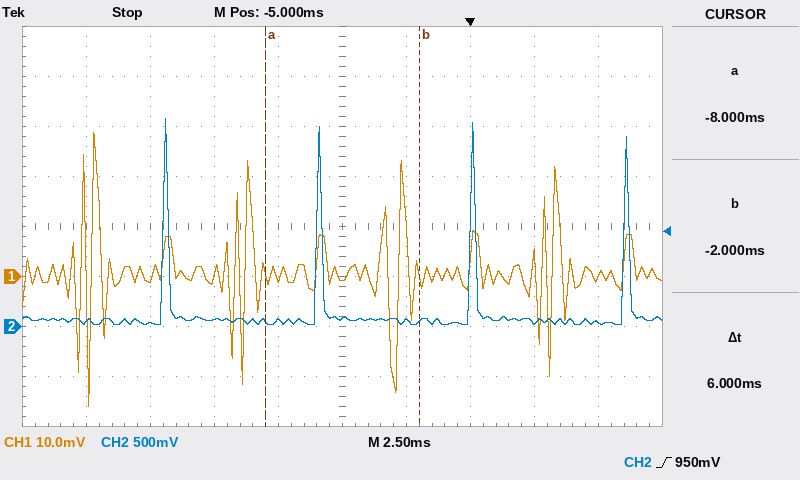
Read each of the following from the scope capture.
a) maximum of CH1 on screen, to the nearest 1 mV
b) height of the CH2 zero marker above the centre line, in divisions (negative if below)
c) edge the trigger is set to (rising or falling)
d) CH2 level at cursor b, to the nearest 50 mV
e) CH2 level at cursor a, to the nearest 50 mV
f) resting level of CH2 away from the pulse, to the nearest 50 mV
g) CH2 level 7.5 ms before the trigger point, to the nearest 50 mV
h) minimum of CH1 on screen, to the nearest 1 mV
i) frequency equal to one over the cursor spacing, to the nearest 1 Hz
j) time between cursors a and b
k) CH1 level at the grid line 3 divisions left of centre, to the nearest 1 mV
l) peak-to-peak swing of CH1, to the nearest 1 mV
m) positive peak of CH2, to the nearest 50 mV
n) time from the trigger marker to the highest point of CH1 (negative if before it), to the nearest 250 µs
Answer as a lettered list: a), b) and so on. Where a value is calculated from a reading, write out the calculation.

a) 29 mV
b) -2.0 div
c) rising
d) 50 mV
e) 50 mV
f) 50 mV
g) 50 mV
h) -26 mV
i) 1 / 6 ms ≈ 167 Hz
j) 6 ms
k) 0 mV
l) 29 mV − (-26 mV) = 55 mV
m) 2.10 V
n) -14.75 ms
